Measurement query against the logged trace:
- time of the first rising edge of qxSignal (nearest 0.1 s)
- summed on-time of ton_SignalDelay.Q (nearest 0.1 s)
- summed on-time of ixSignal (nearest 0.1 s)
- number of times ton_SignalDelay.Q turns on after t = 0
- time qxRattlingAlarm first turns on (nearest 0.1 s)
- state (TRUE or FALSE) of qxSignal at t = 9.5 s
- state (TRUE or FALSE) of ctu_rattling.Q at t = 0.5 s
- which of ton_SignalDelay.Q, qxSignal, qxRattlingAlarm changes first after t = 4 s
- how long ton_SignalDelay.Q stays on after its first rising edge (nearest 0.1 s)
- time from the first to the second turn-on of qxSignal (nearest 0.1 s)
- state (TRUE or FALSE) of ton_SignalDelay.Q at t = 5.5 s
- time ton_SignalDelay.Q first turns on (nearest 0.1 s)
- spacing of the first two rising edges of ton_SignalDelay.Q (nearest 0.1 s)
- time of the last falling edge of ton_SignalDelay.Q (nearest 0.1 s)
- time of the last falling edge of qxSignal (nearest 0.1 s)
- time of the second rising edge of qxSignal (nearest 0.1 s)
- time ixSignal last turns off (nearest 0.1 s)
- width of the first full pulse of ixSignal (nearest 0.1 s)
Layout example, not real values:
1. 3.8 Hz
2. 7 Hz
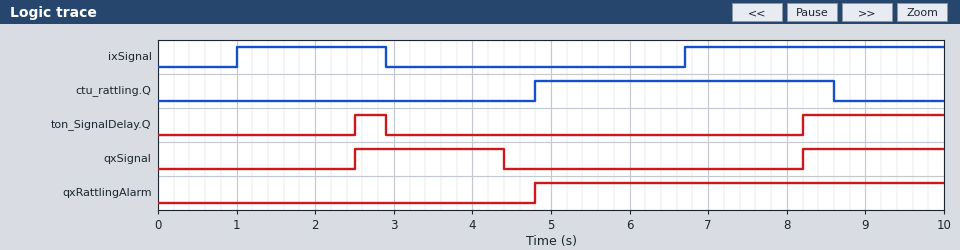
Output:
1. 2.5 s
2. 2.2 s
3. 5.2 s
4. 2
5. 4.8 s
6. TRUE
7. FALSE
8. qxSignal
9. 0.4 s
10. 5.7 s
11. FALSE
12. 2.5 s
13. 5.7 s
14. 2.9 s
15. 4.4 s
16. 8.2 s
17. 2.9 s
18. 1.9 s
